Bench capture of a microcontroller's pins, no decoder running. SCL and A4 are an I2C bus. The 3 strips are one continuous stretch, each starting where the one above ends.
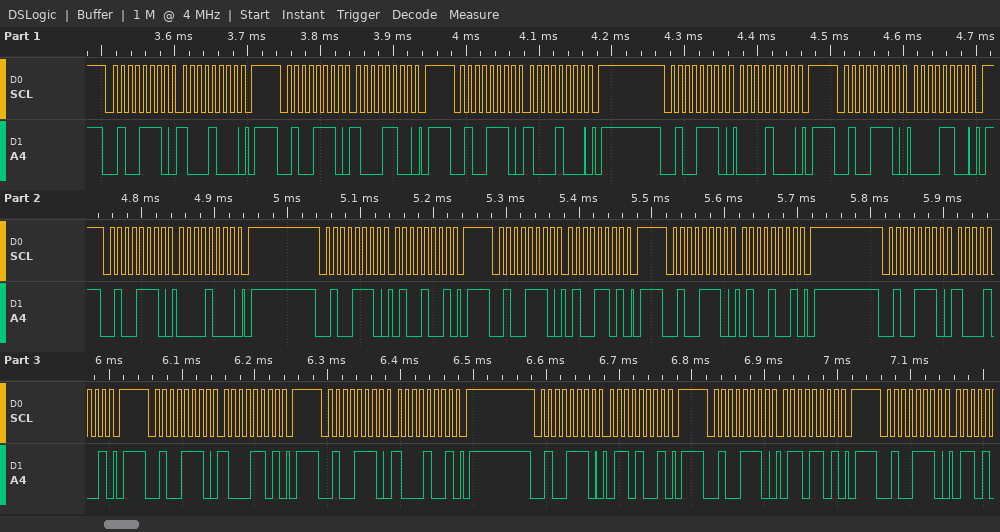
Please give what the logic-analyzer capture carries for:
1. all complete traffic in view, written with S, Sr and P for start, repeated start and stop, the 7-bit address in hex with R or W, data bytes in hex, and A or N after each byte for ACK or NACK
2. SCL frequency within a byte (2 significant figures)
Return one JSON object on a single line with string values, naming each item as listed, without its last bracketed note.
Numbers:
{"all complete traffic in view, written with S, Sr and P for start, repeated start and stop, the 7-bit address in hex with R or W, data bytes in hex, and A or N after each byte for ACK or NACK": "S 27W A 88 A P S 27W A 8C A P S 27W A 88 A P S 27W A 08 A P S 27W A 0C A P S 27W A 08 A P S 27W A 49 A P S 27W A 4D A P S 27W A 49 A P S 27W A 89 A P S 27W A 8D A P S 27W A 89 A P S 27W A 69 A P S 27W A 6D A P S 27W A", "SCL frequency within a byte": "100 kHz"}
